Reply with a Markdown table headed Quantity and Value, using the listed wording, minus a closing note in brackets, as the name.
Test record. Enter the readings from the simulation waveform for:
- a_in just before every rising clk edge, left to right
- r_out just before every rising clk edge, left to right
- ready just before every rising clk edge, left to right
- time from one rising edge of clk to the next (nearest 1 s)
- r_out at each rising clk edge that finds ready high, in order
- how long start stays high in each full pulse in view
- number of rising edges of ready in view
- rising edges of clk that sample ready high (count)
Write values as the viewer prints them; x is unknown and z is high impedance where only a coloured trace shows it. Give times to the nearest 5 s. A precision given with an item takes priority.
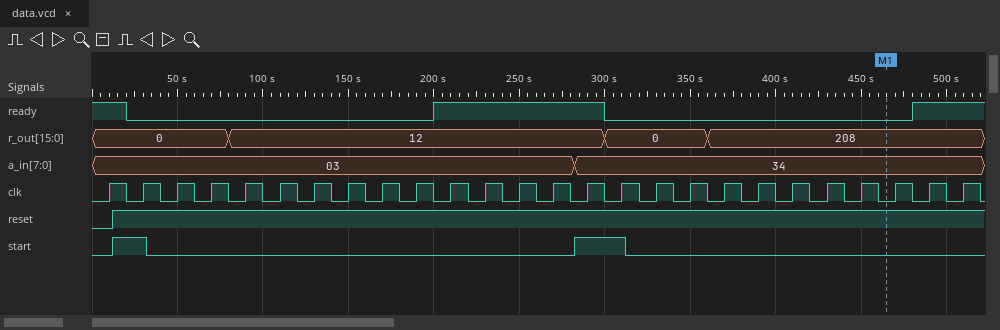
| Quantity | Value |
|---|---|
| a_in just before every rising clk edge, left to right | 03, 03, 03, 03, 03, 03, 03, 03, 03, 03, 03, 03, 03, 03, 34, 34, 34, 34, 34, 34, 34, 34, 34, 34, 34, 34 |
| r_out just before every rising clk edge, left to right | 0, 0, 0, 0, 12, 12, 12, 12, 12, 12, 12, 12, 12, 12, 12, 0, 0, 0, 208, 208, 208, 208, 208, 208, 208, 208 |
| ready just before every rising clk edge, left to right | 1 0 0 0 0 0 0 0 0 0 1 1 1 1 1 0 0 0 0 0 0 0 0 0 1 1 |
| time from one rising edge of clk to the next | 20 s |
| r_out at each rising clk edge that finds ready high, in order | 0, 12, 12, 12, 12, 12, 208, 208 |
| how long start stays high in each full pulse in view | 20 s, 30 s |
| number of rising edges of ready in view | 2 |
| rising edges of clk that sample ready high | 8 |
